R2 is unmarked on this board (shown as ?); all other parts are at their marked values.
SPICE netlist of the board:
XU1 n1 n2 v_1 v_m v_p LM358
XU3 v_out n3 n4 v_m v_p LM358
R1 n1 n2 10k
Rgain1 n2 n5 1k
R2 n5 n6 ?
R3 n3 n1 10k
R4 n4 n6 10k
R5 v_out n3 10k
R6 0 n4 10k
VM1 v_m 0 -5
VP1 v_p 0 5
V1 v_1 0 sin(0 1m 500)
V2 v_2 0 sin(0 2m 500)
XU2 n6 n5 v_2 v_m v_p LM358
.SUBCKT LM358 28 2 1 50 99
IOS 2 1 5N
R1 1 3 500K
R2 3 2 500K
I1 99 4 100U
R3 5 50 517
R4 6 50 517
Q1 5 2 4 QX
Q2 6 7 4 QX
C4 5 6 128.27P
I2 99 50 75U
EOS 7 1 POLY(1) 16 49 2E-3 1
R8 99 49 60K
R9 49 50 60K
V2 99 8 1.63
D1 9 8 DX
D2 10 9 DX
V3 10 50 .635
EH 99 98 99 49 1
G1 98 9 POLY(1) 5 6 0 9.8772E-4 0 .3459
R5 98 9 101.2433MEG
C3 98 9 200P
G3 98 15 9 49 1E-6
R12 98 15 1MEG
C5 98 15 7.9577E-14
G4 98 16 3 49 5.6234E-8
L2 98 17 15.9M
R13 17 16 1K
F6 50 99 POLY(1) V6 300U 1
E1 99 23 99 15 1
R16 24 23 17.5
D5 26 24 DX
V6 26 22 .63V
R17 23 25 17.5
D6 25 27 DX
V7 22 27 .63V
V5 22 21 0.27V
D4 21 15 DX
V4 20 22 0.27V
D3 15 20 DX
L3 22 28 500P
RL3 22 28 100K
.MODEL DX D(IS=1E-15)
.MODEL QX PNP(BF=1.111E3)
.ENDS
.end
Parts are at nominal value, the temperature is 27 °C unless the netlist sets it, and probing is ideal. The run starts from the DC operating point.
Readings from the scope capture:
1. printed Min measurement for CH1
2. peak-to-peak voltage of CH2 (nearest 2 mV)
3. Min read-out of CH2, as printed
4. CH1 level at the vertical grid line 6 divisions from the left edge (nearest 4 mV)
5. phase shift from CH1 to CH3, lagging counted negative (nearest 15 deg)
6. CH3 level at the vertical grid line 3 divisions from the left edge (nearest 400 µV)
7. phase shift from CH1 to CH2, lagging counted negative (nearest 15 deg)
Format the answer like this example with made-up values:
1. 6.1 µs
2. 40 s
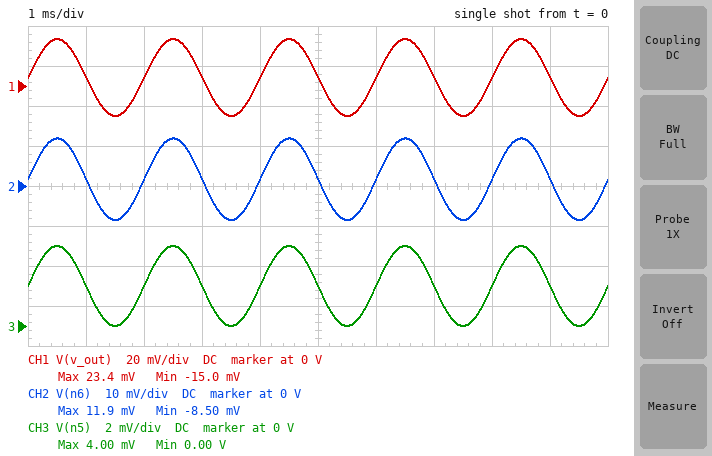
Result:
1. -15.0 mV
2. 20 mV
3. -8.50 mV
4. 4 mV
5. 0 deg
6. 2.0 mV
7. 0 deg
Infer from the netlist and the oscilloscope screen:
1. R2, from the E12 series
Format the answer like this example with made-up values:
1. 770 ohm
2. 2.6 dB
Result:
1. 8.2 kΩ
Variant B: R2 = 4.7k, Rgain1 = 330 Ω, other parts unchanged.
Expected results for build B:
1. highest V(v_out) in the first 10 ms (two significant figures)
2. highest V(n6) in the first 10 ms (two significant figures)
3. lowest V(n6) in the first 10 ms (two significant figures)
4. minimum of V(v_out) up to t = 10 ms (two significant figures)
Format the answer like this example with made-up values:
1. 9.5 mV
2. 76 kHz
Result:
1. 50 mV
2. 18 mV
3. -14 mV
4. -41 mV
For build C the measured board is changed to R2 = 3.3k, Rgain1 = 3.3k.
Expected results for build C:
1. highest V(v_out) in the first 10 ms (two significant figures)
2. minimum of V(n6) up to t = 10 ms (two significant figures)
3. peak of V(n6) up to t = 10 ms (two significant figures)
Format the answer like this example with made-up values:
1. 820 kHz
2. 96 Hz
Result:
1. 9.4 mV
2. -1.1 mV
3. 4.9 mV
